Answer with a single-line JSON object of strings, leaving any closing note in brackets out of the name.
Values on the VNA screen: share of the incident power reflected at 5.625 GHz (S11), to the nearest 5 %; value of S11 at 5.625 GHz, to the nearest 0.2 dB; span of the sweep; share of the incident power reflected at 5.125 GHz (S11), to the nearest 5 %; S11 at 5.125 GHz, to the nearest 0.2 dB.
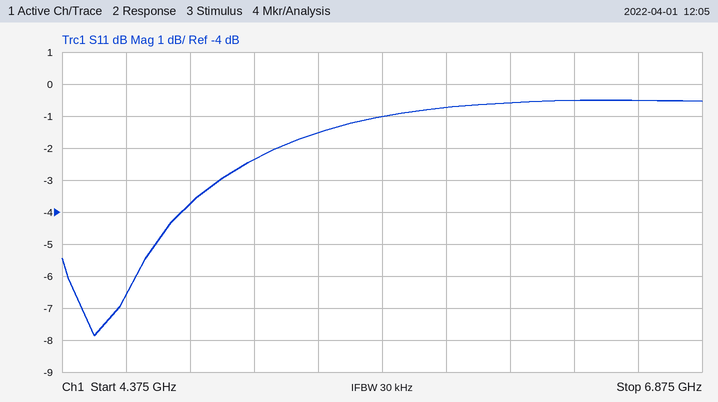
{"share of the incident power reflected at 5.625 GHz (S11), to the nearest 5 %": "80 %", "value of S11 at 5.625 GHz, to the nearest 0.2 dB": "-1.0 dB", "span of the sweep": "2.5 GHz", "share of the incident power reflected at 5.125 GHz (S11), to the nearest 5 %": "60 %", "S11 at 5.125 GHz, to the nearest 0.2 dB": "-2.4 dB"}
